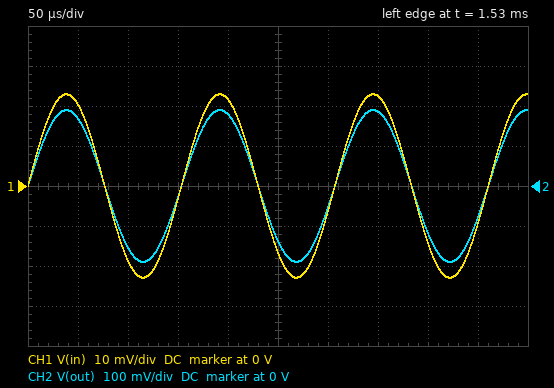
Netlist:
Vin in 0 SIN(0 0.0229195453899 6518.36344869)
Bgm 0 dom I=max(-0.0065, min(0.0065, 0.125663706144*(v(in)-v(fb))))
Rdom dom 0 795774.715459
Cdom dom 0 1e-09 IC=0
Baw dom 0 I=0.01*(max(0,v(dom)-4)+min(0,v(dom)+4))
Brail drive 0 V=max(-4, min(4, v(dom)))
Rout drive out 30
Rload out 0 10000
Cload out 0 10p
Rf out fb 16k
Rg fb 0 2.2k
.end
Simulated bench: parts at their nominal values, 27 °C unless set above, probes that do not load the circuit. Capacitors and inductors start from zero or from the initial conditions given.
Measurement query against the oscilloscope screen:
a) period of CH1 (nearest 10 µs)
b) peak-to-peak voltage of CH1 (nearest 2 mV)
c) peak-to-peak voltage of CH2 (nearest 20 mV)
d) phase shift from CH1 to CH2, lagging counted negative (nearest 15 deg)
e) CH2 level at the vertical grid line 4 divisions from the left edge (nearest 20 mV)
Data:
150 µs
46 mV
380 mV
0 deg
180 mV
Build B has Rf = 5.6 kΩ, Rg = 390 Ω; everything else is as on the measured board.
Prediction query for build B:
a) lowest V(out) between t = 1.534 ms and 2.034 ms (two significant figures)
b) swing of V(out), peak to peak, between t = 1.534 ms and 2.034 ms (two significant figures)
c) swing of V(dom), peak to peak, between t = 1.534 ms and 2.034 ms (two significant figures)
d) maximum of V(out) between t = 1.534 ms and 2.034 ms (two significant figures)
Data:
-350 mV
700 mV
710 mV
350 mV
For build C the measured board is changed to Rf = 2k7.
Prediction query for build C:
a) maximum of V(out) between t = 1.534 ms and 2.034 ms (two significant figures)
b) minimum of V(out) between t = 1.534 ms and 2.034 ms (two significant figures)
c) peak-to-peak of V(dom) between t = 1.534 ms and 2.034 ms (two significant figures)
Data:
51 mV
-51 mV
100 mV
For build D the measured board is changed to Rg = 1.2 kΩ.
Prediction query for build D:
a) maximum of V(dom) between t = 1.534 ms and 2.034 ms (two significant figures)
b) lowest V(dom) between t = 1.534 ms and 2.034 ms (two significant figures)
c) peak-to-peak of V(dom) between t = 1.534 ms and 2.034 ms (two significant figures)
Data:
330 mV
-330 mV
660 mV
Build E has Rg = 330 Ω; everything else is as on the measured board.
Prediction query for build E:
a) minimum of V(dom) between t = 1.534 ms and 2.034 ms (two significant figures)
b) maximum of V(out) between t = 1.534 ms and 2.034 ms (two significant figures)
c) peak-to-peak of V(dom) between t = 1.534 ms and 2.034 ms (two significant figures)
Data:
-1.1 V
1.1 V
2.3 V
